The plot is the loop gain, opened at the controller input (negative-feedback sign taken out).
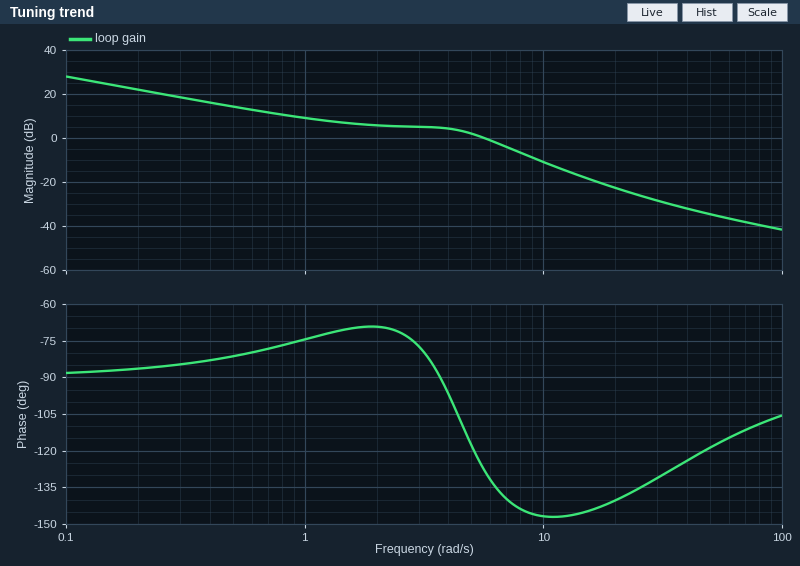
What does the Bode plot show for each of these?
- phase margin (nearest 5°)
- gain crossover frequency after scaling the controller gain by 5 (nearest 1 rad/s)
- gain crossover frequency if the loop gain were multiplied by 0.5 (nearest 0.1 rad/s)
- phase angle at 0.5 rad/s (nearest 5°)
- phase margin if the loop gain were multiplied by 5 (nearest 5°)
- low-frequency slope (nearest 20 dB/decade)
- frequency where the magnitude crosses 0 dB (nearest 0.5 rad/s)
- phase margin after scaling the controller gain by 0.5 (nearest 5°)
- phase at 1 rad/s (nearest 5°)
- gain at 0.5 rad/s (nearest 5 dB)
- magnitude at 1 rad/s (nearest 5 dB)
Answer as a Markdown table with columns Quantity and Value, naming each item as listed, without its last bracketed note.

| Quantity | Value |
|---|---|
| phase margin | 50° |
| gain crossover frequency after scaling the controller gain by 5 | 12 rad/s |
| gain crossover frequency if the loop gain were multiplied by 0.5 | 1.8 rad/s |
| phase angle at 0.5 rad/s | -80° |
| phase margin if the loop gain were multiplied by 5 | 35° |
| low-frequency slope | -20 dB/decade |
| frequency where the magnitude crosses 0 dB | 5.5 rad/s |
| phase margin after scaling the controller gain by 0.5 | 110° |
| phase at 1 rad/s | -75° |
| gain at 0.5 rad/s | 15 dB |
| magnitude at 1 rad/s | 10 dB |
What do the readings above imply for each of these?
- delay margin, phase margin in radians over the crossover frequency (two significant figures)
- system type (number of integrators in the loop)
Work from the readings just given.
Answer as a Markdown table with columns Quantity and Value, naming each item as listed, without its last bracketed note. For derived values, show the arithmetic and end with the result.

| Quantity | Value |
|---|---|
| delay margin, phase margin in radians over the crossover frequency | 50 × π / 180 / 5.5 = 0.16 s |
| system type | 1 |
